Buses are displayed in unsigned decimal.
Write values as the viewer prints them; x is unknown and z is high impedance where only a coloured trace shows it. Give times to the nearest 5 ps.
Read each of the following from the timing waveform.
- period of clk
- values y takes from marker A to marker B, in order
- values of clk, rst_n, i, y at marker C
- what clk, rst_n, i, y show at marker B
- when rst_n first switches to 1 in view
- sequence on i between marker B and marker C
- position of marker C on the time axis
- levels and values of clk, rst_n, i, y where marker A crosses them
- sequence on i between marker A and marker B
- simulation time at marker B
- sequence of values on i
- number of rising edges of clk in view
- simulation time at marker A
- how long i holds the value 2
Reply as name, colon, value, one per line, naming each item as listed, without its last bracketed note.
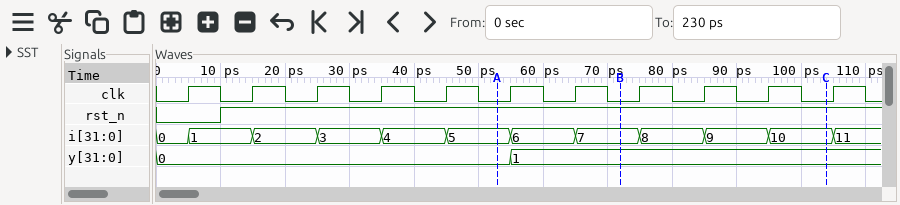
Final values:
period of clk: 10 ps
values y takes from marker A to marker B, in order: 0, 1
values of clk, rst_n, i, y at marker C: clk=0, rst_n=1, i=10, y=1
what clk, rst_n, i, y show at marker B: clk=0, rst_n=1, i=7, y=1
when rst_n first switches to 1 in view: 10 ps
sequence on i between marker B and marker C: 7, 8, 9, 10
position of marker C on the time axis: 105 ps
levels and values of clk, rst_n, i, y where marker A crosses them: clk=0, rst_n=1, i=5, y=0
sequence on i between marker A and marker B: 5, 6, 7
simulation time at marker B: 70 ps
sequence of values on i: 0, 1, 2, 3, 4, 5, 6, 7, 8, 9, 10, 11
number of rising edges of clk in view: 11
simulation time at marker A: 55 ps
how long i holds the value 2: 10 ps
